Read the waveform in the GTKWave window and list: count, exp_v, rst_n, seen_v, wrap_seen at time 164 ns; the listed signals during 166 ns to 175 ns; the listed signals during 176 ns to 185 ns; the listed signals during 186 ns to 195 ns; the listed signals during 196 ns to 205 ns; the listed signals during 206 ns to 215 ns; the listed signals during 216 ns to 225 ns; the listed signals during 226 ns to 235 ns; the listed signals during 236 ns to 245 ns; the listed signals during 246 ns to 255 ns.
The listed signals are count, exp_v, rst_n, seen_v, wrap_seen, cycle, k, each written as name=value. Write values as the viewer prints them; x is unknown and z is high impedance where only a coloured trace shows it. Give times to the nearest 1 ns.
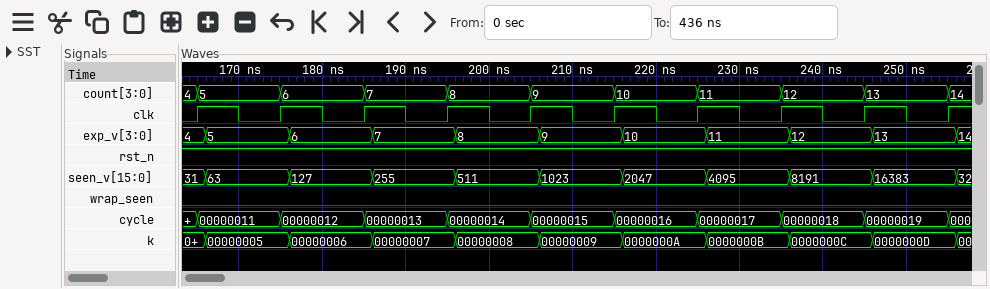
count=4, exp_v=4, rst_n=1, seen_v=31, wrap_seen=0
count=5, exp_v=5, rst_n=1, seen_v=63, wrap_seen=0, cycle=00000011, k=00000005
count=6, exp_v=6, rst_n=1, seen_v=127, wrap_seen=0, cycle=00000012, k=00000006
count=7, exp_v=7, rst_n=1, seen_v=255, wrap_seen=0, cycle=00000013, k=00000007
count=8, exp_v=8, rst_n=1, seen_v=511, wrap_seen=0, cycle=00000014, k=00000008
count=9, exp_v=9, rst_n=1, seen_v=1023, wrap_seen=0, cycle=00000015, k=00000009
count=10, exp_v=10, rst_n=1, seen_v=2047, wrap_seen=0, cycle=00000016, k=0000000A
count=11, exp_v=11, rst_n=1, seen_v=4095, wrap_seen=0, cycle=00000017, k=0000000B
count=12, exp_v=12, rst_n=1, seen_v=8191, wrap_seen=0, cycle=00000018, k=0000000C
count=13, exp_v=13, rst_n=1, seen_v=16383, wrap_seen=0, cycle=00000019, k=0000000D
